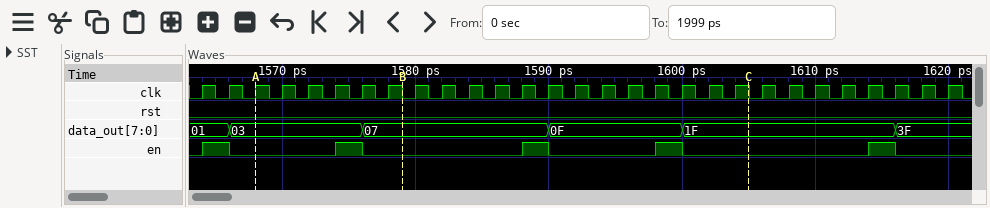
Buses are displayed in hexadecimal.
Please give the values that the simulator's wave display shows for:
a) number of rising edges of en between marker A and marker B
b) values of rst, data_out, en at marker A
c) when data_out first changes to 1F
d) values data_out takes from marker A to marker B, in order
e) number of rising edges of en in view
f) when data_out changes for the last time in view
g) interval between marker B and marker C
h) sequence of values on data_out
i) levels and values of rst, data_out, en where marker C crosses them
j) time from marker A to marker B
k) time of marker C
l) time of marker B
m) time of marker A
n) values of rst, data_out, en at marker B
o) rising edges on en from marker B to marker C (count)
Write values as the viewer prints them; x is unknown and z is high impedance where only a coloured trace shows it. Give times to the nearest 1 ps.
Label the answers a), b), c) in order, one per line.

a) 1
b) rst=0, data_out=03, en=0
c) 1600 ps
d) 03, 07
e) 5
f) 1616 ps
g) 26 ps
h) 01, 03, 07, 0F, 1F, 3F
i) rst=0, data_out=1F, en=0
j) 11 ps
k) 1605 ps
l) 1579 ps
m) 1568 ps
n) rst=0, data_out=07, en=0
o) 2
